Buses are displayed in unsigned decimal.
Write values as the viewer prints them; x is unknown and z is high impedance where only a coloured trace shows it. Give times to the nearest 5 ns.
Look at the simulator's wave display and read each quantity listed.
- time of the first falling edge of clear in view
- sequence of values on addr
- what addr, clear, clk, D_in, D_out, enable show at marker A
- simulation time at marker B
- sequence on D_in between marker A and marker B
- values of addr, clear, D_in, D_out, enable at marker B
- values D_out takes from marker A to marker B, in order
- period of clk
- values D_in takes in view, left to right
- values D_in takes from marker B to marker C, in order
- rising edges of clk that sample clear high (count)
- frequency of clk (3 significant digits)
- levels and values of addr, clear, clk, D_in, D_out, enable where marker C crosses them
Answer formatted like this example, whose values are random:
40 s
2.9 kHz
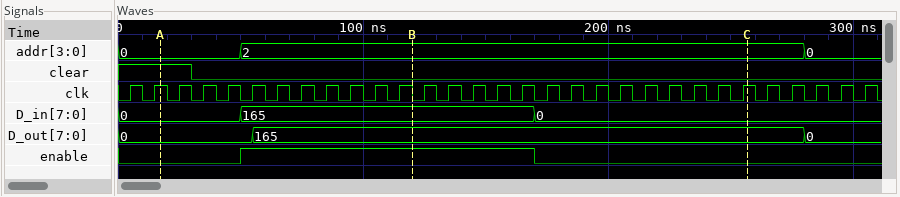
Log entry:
30 ns
0, 2, 0
addr=0, clear=1, clk=1, D_in=0, D_out=0, enable=0
120 ns
0, 165
addr=2, clear=0, D_in=165, D_out=165, enable=1
0, 165
10 ns
0, 165, 0
165, 0
3
100 MHz
addr=2, clear=0, clk=1, D_in=0, D_out=165, enable=0
